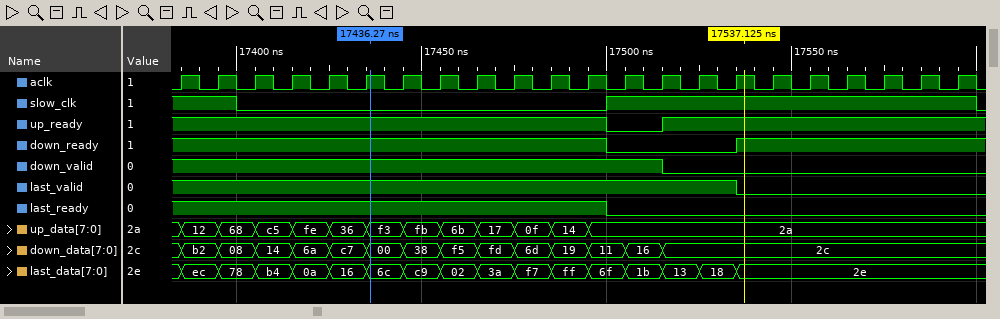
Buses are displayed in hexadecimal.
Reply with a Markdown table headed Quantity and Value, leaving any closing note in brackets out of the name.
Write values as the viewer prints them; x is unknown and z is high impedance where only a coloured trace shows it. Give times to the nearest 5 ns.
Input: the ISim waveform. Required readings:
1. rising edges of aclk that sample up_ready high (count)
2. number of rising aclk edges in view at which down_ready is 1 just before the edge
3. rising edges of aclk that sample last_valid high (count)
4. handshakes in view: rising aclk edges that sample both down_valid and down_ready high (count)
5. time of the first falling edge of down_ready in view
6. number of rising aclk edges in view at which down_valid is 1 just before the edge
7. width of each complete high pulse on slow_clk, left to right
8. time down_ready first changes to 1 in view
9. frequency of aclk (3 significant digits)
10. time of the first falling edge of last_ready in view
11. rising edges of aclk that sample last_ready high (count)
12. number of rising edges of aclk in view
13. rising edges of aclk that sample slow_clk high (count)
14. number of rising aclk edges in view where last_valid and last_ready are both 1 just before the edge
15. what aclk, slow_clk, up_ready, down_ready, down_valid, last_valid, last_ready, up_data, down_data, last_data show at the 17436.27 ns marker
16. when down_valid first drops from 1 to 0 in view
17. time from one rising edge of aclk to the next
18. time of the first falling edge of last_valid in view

| Quantity | Value |
|---|---|
| rising edges of aclk that sample up_ready high | 20 |
| number of rising aclk edges in view at which down_ready is 1 just before the edge | 18 |
| rising edges of aclk that sample last_valid high | 16 |
| handshakes in view: rising aclk edges that sample both down_valid and down_ready high | 12 |
| time of the first falling edge of down_ready in view | 17500 ns |
| number of rising aclk edges in view at which down_valid is 1 just before the edge | 14 |
| width of each complete high pulse on slow_clk, left to right | 100 ns |
| time down_ready first changes to 1 in view | 17535 ns |
| frequency of aclk | 100 MHz |
| time of the first falling edge of last_ready in view | 17500 ns |
| rising edges of aclk that sample last_ready high | 12 |
| number of rising edges of aclk in view | 22 |
| rising edges of aclk that sample slow_clk high | 12 |
| number of rising aclk edges in view where last_valid and last_ready are both 1 just before the edge | 12 |
| what aclk, slow_clk, up_ready, down_ready, down_valid, last_valid, last_ready, up_data, down_data, last_data show at the 17436.27 ns marker | aclk=1, slow_clk=0, up_ready=1, down_ready=1, down_valid=1, last_valid=1, last_ready=1, up_data=f3, down_data=00, last_data=6c |
| when down_valid first drops from 1 to 0 in view | 17515 ns |
| time from one rising edge of aclk to the next | 10 ns |
| time of the first falling edge of last_valid in view | 17535 ns |
